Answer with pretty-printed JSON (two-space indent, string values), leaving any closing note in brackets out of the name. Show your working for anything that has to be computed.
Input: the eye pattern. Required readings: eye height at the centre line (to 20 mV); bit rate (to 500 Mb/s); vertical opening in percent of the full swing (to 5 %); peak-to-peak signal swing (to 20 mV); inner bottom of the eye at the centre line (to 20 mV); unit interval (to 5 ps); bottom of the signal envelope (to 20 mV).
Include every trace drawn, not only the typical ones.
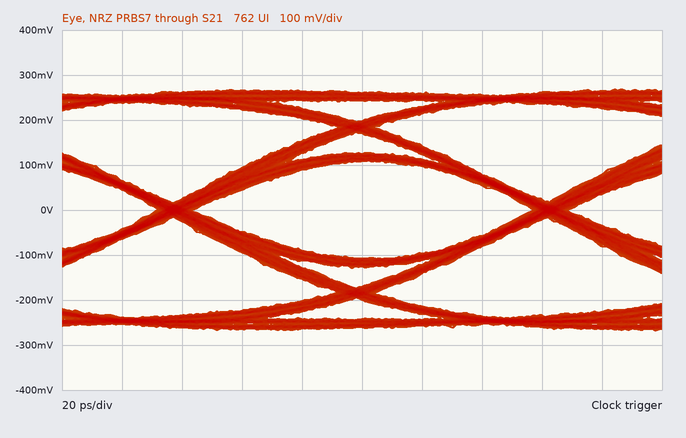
{
  "eye height at the centre line": "220 mV",
  "bit rate": "8.0 Gb/s",
  "vertical opening in percent of the full swing": "220 mV / 540 mV ≈ 40.7 %, so 40 % to the nearest 5 %",
  "peak-to-peak signal swing": "540 mV",
  "inner bottom of the eye at the centre line": "-100 mV",
  "unit interval": "125 ps",
  "bottom of the signal envelope": "-260 mV"
}
